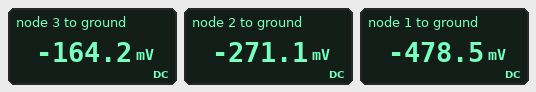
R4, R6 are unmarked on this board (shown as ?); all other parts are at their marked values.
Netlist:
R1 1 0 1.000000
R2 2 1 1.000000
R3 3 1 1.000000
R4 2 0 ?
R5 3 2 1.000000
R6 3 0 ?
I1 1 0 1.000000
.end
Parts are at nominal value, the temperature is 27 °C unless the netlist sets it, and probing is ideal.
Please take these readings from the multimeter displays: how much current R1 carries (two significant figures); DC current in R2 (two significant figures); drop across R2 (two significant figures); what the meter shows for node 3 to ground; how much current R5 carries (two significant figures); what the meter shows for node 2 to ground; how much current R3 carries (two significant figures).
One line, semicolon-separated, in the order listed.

480 mA; 210 mA; 210 mV; -164.2 mV; 110 mA; -271.1 mV; 310 mA
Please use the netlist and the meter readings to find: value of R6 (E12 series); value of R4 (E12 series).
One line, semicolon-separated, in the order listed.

0.39 Ω; 2.7 Ω
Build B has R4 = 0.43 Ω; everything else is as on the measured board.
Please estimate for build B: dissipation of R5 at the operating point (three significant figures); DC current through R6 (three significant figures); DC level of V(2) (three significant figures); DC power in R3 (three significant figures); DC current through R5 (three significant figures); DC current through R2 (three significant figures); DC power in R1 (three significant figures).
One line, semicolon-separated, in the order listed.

27.7 µW; 301 mA; -123 mV; 87.6 mW; 5.26 mA; 291 mA; 171 mW
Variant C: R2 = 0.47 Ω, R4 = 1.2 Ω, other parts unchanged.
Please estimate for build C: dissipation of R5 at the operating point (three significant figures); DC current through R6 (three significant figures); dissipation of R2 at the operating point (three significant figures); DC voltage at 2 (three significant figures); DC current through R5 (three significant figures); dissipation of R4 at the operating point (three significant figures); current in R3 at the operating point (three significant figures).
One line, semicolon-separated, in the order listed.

12.3 mW; 375 mA; 49.8 mW; -257 mV; 111 mA; 55.2 mW; 264 mA
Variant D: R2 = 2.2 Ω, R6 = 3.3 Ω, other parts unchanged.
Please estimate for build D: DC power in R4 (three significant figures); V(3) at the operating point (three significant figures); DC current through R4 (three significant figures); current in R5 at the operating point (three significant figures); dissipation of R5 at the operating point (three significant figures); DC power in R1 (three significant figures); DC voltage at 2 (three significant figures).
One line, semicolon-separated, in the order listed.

71.7 mW; -490 mV; 163 mA; 50.0 mA; 2.50 mW; 474 mW; -440 mV
